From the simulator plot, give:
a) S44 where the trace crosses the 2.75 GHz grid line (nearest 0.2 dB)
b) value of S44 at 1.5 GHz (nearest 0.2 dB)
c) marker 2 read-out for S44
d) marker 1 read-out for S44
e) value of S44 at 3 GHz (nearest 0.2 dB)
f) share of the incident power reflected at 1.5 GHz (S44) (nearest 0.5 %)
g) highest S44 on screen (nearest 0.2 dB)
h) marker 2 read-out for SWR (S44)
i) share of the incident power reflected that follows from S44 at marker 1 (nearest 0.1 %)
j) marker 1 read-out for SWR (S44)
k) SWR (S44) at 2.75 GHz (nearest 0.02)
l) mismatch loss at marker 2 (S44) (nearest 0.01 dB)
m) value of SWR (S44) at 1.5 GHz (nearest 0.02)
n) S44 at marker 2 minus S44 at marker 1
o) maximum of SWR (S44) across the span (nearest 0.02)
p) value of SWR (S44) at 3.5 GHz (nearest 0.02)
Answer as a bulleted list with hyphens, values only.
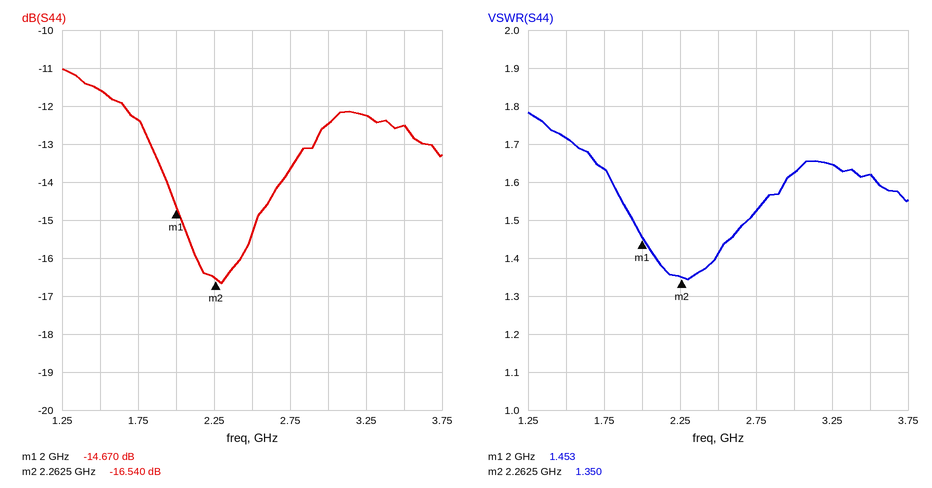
- -13.6 dB
- -11.6 dB
- -16.540 dB
- -14.670 dB
- -12.4 dB
- 7.0 %
- -11.0 dB
- 1.350
- 3.4 %
- 1.453
- 1.52
- 0.10 dB
- 1.72
- -1.870 dB
- 1.78
- 1.62
